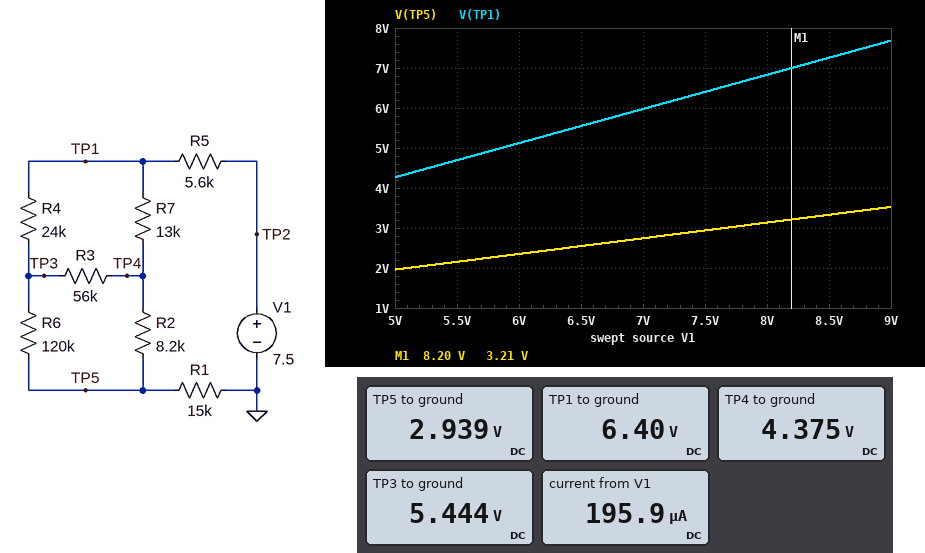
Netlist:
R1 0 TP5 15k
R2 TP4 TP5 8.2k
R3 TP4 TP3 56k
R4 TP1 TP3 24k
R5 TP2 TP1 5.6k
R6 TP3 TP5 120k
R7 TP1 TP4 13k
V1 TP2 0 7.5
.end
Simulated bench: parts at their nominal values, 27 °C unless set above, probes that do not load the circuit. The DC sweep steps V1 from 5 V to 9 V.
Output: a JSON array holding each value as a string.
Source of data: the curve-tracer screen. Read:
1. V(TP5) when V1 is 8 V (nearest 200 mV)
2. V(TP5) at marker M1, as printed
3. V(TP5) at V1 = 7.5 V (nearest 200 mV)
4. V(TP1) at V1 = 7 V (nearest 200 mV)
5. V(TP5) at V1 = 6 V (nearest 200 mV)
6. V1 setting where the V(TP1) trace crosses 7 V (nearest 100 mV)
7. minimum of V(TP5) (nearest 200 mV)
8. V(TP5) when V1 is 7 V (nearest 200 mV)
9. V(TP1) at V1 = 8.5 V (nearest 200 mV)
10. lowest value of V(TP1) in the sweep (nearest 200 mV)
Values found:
["3.2 V", "3.21 V", "3.0 V", "6.0 V", "2.4 V", "8.2 V", "2.0 V", "2.8 V", "7.2 V", "4.2 V"]
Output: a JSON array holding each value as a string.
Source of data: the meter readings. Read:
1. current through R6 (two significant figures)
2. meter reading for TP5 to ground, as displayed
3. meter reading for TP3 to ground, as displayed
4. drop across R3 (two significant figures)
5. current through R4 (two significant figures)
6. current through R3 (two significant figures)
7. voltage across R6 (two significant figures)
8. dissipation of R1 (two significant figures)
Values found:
["21 µA", "2.939 V", "5.444 V", "1.1 V", "40 µA", "19 µA", "2.5 V", "580 µW"]
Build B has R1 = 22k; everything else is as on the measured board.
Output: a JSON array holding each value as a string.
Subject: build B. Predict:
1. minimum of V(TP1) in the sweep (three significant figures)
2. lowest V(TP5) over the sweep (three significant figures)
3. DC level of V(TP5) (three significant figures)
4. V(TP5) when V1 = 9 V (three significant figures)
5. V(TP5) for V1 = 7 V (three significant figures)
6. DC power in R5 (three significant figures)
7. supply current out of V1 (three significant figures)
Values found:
["4.38 V", "2.43 V", "3.64 V", "4.37 V", "3.40 V", "154 µW", "166 µA"]
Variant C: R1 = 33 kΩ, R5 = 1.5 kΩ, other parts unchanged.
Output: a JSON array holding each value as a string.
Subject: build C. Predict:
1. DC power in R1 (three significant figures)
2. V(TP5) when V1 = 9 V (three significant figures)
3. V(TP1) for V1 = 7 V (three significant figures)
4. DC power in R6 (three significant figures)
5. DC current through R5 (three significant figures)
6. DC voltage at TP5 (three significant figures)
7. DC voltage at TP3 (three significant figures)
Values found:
["682 µW", "5.69 V", "6.80 V", "28.1 µW", "144 µA", "4.74 V", "6.58 V"]
